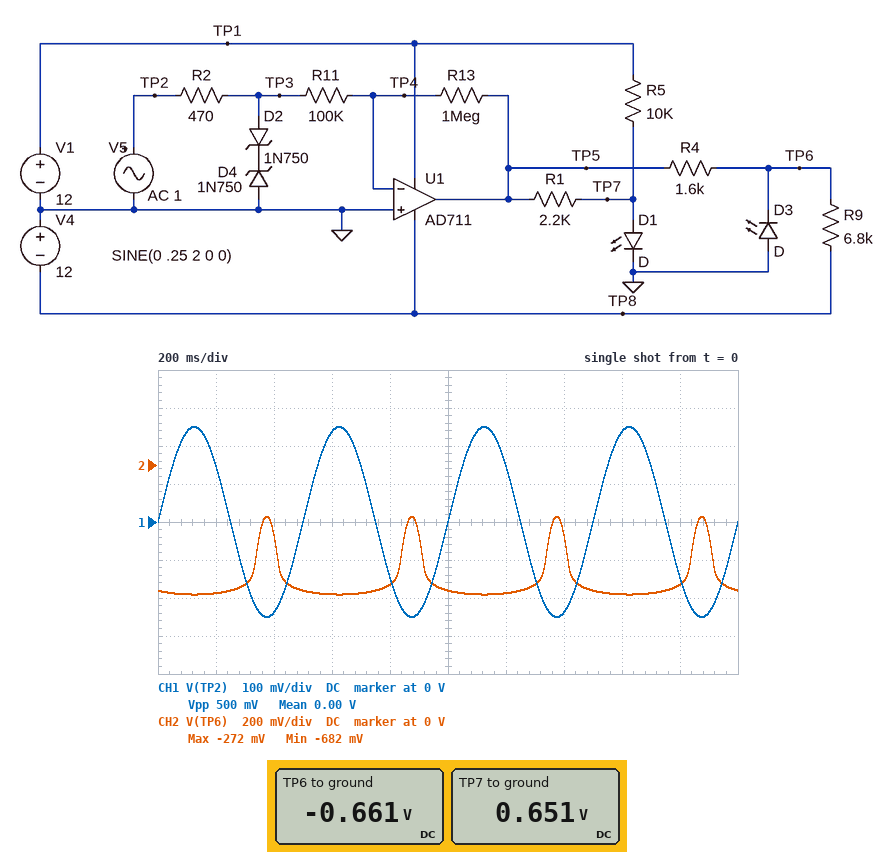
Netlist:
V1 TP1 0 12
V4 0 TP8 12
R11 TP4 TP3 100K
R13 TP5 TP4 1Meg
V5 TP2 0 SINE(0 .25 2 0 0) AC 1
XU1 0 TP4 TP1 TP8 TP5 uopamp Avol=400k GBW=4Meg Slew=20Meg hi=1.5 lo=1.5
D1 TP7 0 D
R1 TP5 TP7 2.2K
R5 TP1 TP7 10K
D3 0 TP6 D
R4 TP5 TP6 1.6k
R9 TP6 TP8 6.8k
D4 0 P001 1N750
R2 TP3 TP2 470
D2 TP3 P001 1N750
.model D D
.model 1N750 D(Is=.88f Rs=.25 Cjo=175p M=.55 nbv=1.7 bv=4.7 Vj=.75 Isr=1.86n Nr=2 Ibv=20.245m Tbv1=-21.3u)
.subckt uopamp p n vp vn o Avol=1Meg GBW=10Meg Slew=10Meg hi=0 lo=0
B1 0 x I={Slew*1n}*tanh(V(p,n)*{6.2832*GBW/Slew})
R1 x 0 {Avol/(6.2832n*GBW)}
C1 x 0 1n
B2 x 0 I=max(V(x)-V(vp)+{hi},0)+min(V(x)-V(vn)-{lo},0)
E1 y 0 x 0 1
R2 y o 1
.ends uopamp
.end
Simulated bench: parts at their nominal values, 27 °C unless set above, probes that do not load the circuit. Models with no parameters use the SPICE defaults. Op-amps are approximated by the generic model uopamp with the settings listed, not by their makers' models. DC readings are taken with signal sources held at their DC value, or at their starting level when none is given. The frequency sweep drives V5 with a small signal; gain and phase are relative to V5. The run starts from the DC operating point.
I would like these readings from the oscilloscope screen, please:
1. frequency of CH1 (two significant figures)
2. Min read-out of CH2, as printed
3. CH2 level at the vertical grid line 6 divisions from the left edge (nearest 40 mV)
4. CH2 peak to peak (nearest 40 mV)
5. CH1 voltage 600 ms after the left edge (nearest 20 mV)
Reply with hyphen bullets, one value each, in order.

- 2.0 Hz
- -682 mV
- -680 mV
- 400 mV
- 240 mV
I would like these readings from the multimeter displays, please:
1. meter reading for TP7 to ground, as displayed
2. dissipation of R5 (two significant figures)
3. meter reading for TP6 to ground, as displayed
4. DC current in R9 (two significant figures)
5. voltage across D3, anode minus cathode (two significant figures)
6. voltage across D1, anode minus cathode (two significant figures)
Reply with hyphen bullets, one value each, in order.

- 0.651 V
- 13 mW
- -0.661 V
- 1.7 mA
- 660 mV
- 650 mV
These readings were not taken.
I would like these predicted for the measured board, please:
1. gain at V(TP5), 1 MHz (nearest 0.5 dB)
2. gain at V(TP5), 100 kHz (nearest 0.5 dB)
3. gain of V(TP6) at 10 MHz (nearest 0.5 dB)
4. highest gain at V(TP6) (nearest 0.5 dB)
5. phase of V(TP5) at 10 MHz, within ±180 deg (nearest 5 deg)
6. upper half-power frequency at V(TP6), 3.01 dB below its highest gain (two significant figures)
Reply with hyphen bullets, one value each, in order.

- 10.5 dB
- 19.5 dB
- -55.5 dB
- -18.0 dB
- 25 deg
- 360 kHz
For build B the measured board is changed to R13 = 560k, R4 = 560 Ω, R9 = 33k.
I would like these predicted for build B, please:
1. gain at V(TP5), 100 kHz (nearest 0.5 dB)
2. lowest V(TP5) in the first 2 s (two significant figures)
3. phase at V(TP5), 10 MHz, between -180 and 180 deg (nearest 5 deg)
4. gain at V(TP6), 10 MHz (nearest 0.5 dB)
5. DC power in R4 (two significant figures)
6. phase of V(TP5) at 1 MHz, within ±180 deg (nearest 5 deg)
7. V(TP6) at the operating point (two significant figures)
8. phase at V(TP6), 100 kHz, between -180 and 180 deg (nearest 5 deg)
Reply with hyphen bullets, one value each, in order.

- 15.0 dB
- -1.4 V
- 25 deg
- -18.5 dB
- 72 µW
- 105 deg
- -200 mV
- 170 deg
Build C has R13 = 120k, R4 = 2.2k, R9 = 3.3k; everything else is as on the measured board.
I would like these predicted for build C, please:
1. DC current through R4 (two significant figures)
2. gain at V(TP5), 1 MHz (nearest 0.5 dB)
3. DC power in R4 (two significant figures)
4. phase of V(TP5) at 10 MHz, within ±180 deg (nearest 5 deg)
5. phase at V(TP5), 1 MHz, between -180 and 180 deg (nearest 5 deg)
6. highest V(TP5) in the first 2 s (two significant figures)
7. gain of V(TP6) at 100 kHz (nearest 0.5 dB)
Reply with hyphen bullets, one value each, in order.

- 310 µA
- 0 dB
- 210 µW
- 30 deg
- 135 deg
- 300 mV
- -47.0 dB
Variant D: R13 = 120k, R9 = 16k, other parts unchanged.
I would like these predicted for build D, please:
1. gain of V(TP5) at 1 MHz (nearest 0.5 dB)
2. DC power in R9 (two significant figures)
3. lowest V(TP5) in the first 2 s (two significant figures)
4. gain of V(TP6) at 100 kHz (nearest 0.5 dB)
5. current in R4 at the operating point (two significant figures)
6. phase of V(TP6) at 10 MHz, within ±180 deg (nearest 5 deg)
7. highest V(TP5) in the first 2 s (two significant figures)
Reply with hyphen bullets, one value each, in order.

- 0 dB
- 8.1 mW
- -300 mV
- -25.0 dB
- 390 µA
- 30 deg
- 300 mV
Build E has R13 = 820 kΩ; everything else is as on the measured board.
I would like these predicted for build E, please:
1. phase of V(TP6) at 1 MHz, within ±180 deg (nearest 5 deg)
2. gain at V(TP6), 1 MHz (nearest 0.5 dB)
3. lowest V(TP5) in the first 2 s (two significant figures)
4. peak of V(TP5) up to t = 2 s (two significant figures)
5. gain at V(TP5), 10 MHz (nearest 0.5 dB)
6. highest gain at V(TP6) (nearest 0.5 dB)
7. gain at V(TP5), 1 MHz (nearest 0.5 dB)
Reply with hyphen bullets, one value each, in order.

- 100 deg
- -28.0 dB
- -2.0 V
- 2.0 V
- -18.0 dB
- -19.5 dB
- 10.0 dB
